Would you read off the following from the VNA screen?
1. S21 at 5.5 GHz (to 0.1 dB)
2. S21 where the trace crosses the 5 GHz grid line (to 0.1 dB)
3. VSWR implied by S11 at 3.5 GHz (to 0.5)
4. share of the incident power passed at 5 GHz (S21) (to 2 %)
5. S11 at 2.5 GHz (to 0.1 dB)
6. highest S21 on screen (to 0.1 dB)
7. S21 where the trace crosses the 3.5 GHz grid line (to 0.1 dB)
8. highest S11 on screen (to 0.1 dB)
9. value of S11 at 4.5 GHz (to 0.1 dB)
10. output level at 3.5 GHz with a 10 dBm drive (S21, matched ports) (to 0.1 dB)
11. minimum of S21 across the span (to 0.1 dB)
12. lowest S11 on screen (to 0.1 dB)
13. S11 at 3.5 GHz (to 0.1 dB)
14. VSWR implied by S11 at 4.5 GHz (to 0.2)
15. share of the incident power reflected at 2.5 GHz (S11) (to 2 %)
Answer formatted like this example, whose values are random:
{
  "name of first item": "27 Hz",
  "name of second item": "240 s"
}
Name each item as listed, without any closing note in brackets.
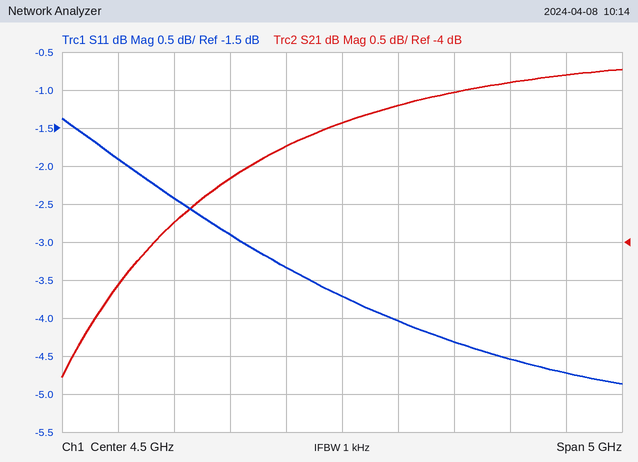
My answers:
{
  "S21 at 5.5 GHz": "-2.0 dB",
  "S21 where the trace crosses the 5 GHz grid line": "-2.2 dB",
  "VSWR implied by S11 at 3.5 GHz": "6.0",
  "share of the incident power passed at 5 GHz (S21)": "60 %",
  "S11 at 2.5 GHz": "-1.9 dB",
  "highest S21 on screen": "-1.7 dB",
  "S21 where the trace crosses the 3.5 GHz grid line": "-3.2 dB",
  "highest S11 on screen": "-1.4 dB",
  "value of S11 at 4.5 GHz": "-3.7 dB",
  "output level at 3.5 GHz with a 10 dBm drive (S21, matched ports)": "6.8 dBm",
  "minimum of S21 across the span": "-5.8 dB",
  "lowest S11 on screen": "-4.9 dB",
  "S11 at 3.5 GHz": "-2.9 dB",
  "VSWR implied by S11 at 4.5 GHz": "4.8",
  "share of the incident power reflected at 2.5 GHz (S11)": "64 %"
}
